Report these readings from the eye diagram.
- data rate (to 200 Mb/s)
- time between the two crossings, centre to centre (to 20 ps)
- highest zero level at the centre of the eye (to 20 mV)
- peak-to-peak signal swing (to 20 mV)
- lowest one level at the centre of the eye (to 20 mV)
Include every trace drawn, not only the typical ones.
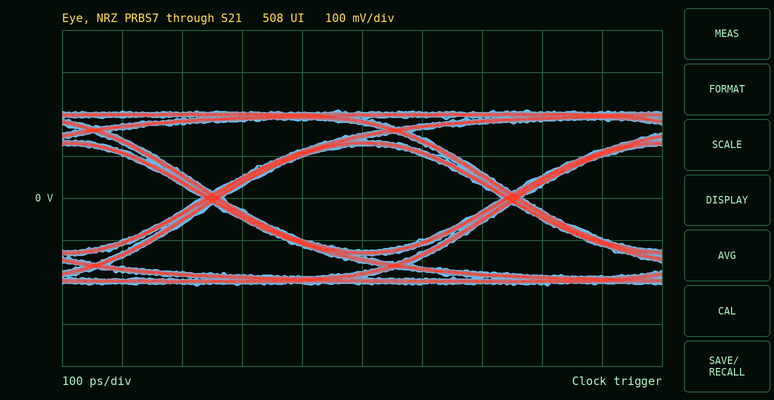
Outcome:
2.0 Gb/s
500 ps
-120 mV
420 mV
120 mV
